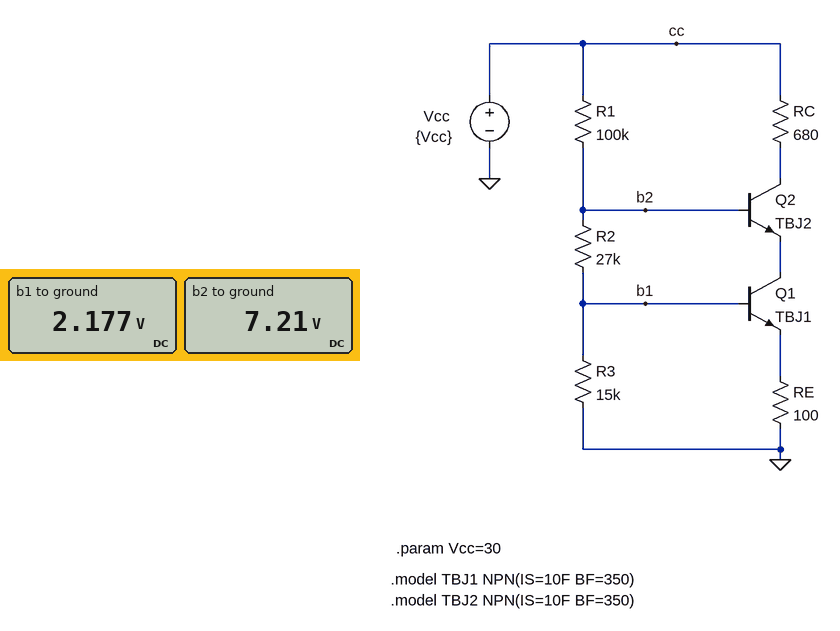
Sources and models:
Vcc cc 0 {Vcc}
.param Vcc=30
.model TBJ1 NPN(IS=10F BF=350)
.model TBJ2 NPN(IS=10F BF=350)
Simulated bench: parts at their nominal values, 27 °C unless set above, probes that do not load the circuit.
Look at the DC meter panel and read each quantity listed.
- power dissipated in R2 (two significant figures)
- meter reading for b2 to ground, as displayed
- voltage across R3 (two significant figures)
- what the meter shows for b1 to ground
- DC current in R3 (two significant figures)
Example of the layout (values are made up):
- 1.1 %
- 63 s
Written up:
- 940 µW
- 7.21 V
- 2.2 V
- 2.177 V
- 150 µA
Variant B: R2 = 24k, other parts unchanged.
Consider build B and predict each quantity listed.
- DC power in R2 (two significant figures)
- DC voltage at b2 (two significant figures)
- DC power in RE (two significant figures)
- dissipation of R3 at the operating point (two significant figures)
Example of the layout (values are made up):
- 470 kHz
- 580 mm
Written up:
- 870 µW
- 6.8 V
- 22 mW
- 330 µW
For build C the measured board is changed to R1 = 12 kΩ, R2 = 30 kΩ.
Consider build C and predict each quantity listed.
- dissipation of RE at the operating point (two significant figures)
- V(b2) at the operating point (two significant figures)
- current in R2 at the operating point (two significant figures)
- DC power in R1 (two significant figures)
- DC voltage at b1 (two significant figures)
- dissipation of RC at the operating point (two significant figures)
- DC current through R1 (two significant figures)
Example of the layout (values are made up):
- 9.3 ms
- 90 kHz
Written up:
- 75 mW
- 13 V
- 310 µA
- 25 mW
- 3.5 V
- 470 mW
- 1.4 mA
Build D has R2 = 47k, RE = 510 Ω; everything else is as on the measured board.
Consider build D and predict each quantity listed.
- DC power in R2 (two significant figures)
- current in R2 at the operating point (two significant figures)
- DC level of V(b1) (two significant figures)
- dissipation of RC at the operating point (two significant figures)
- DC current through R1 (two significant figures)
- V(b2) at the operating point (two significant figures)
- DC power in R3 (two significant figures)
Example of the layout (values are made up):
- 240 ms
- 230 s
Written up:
- 1.5 mW
- 180 µA
- 2.5 V
- 8.9 mW
- 190 µA
- 11 V
- 430 µW
